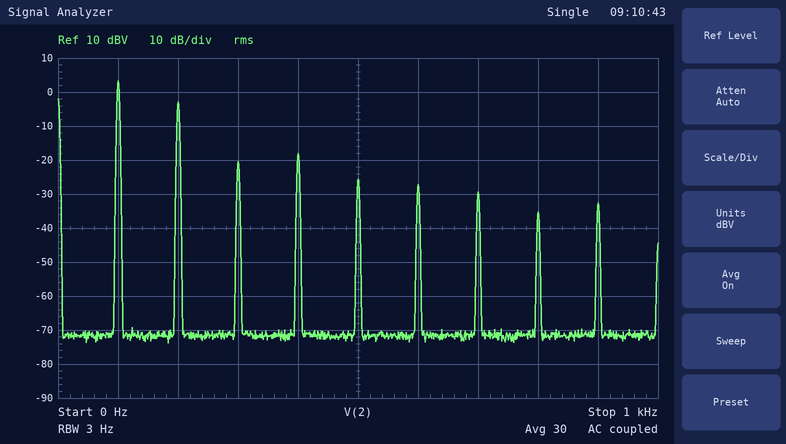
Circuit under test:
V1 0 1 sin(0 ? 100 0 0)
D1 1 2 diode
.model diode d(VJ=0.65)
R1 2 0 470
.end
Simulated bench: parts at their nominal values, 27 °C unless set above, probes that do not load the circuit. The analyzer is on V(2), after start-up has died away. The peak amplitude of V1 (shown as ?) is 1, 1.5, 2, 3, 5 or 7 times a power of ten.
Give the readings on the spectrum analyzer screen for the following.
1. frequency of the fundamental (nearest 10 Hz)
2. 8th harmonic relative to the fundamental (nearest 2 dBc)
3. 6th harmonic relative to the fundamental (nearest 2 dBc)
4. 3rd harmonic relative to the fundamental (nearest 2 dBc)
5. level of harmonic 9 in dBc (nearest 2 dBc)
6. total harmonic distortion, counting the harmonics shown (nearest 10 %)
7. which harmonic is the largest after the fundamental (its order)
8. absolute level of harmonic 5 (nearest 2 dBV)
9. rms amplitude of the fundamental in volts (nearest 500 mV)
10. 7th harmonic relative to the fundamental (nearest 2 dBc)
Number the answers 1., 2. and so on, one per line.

1. 100 Hz
2. -38 dBc
3. -30 dBc
4. -24 dBc
5. -36 dBc
6. 50 %
7. 2
8. -26 dBV
9. 1.5 V
10. -32 dBc
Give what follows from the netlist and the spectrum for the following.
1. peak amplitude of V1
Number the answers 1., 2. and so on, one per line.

1. 5 V
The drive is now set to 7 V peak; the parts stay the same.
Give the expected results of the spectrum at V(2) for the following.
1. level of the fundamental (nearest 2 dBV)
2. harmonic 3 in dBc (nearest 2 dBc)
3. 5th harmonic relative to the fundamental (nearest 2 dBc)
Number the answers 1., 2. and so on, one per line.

1. 6 dBV
2. -26 dBc
3. -32 dBc
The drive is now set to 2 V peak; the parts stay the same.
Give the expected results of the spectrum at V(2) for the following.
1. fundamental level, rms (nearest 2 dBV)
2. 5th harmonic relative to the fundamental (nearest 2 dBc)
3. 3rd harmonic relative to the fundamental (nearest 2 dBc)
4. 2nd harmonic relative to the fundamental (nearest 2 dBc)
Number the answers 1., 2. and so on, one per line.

1. -8 dBV
2. -22 dBc
3. -14 dBc
4. -4 dBc
